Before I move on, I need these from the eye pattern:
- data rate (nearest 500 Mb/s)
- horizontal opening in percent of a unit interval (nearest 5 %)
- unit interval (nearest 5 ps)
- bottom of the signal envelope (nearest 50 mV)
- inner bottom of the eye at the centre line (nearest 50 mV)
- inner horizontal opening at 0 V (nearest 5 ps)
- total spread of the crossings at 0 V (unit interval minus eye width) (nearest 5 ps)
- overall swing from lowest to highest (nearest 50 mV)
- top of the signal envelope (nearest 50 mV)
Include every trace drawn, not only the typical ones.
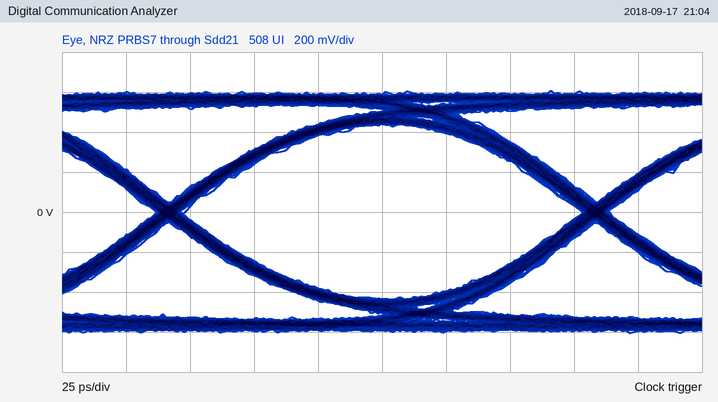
6.0 Gb/s
95 %
165 ps
-600 mV
-450 mV
155 ps
10 ps
1.20 V
600 mV
